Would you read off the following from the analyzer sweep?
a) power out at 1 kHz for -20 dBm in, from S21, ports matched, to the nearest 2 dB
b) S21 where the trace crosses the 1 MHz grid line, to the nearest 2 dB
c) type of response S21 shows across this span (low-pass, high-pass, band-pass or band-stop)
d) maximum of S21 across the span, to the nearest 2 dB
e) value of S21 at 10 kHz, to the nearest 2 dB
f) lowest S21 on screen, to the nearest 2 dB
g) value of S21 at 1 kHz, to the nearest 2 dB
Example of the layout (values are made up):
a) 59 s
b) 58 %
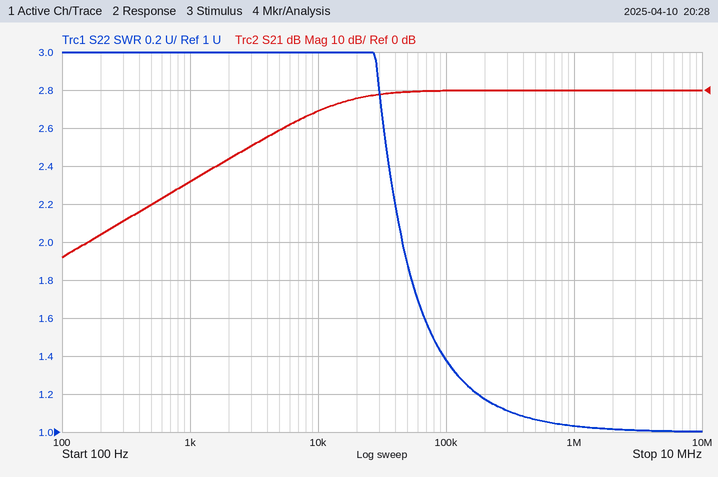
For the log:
a) -44 dBm
b) 0 dB
c) high-pass
d) 0 dB
e) -6 dB
f) -44 dB
g) -24 dB
